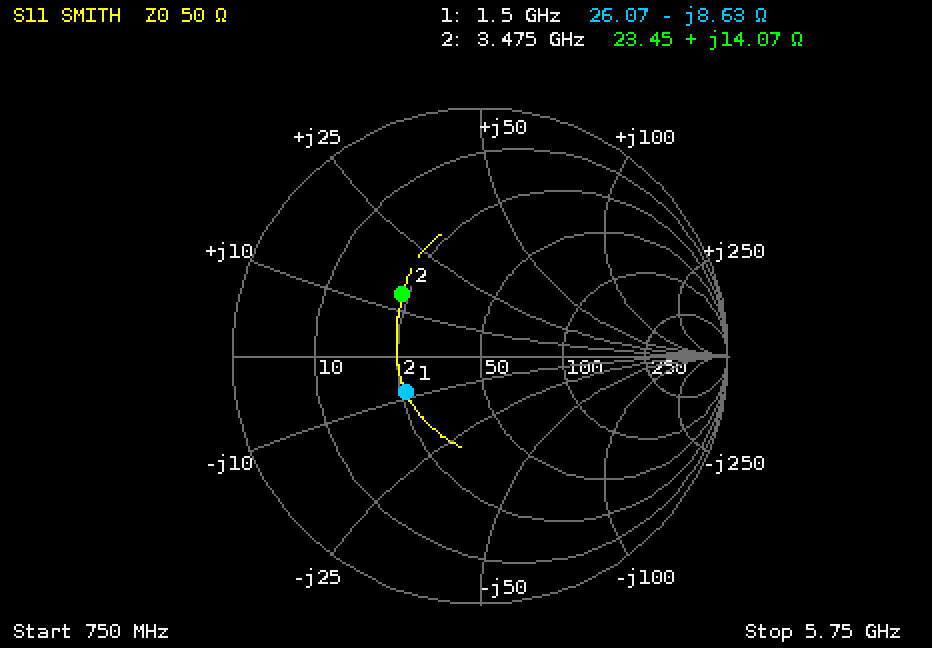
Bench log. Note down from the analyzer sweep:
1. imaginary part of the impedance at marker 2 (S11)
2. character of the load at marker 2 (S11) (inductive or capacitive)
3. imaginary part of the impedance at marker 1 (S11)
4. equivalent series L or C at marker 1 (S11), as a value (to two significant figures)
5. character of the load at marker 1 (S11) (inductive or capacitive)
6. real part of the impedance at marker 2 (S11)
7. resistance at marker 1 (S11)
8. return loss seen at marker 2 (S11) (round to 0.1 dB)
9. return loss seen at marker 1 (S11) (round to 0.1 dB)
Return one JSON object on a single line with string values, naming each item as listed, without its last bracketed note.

{"imaginary part of the impedance at marker 2": "+14.07 Ω", "character of the load at marker 2 (S11)": "inductive", "imaginary part of the impedance at marker 1": "-8.63 Ω", "equivalent series L or C at marker 1 (S11), as a value": "12 pF", "character of the load at marker 1 (S11)": "capacitive", "real part of the impedance at marker 2": "23.45 Ω", "resistance at marker 1": "26.07 Ω", "return loss seen at marker 2 (S11)": "7.9 dB", "return loss seen at marker 1 (S11)": "9.6 dB"}
